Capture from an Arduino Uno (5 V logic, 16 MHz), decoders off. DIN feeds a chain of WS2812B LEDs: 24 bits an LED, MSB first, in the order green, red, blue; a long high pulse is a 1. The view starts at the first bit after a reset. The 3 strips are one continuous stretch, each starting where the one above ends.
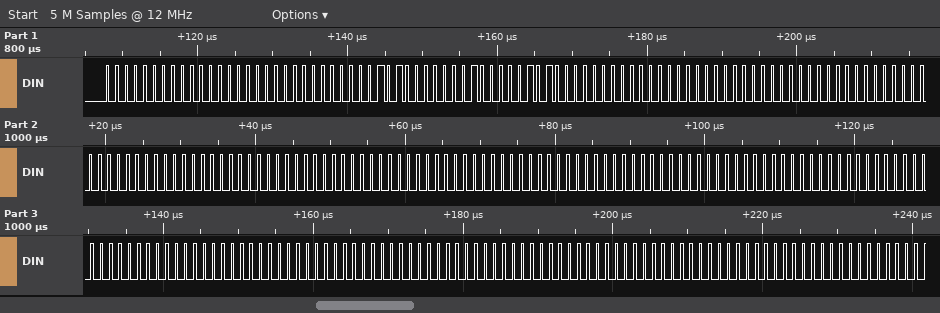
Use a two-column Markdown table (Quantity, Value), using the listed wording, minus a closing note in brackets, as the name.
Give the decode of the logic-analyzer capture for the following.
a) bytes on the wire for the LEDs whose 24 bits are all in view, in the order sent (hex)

| Quantity | Value |
|---|---|
| bytes on the wire for the LEDs whose 24 bits are all in view, in the order sent | 00 00 00 05 01 05 00 00 00 00 00 00 00 00 00 00 00 00 00 00 00 00 00 00 00 00 00 00 00 00 00 00 00 |
